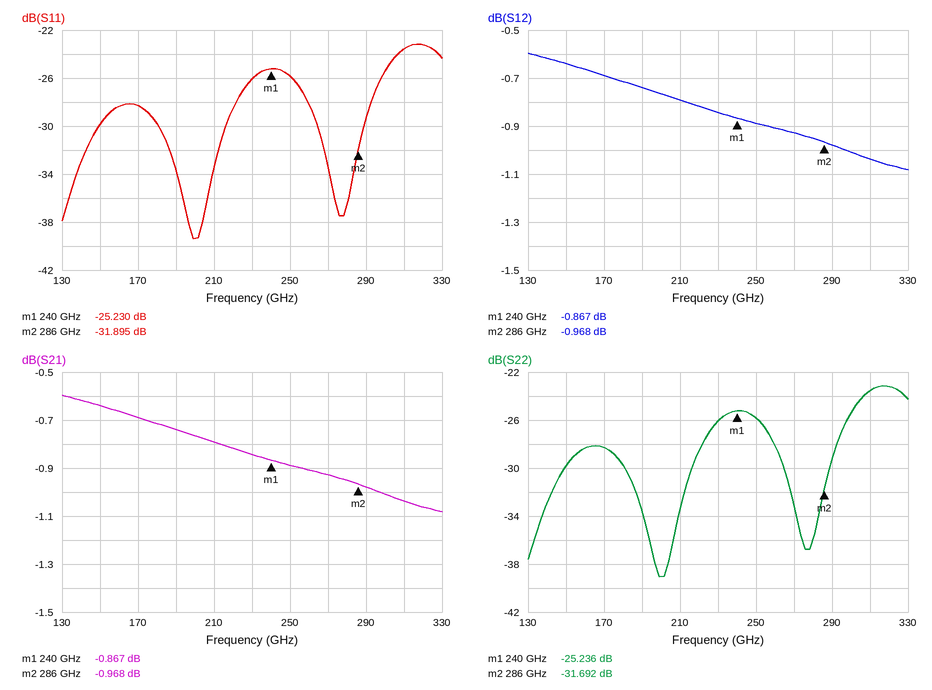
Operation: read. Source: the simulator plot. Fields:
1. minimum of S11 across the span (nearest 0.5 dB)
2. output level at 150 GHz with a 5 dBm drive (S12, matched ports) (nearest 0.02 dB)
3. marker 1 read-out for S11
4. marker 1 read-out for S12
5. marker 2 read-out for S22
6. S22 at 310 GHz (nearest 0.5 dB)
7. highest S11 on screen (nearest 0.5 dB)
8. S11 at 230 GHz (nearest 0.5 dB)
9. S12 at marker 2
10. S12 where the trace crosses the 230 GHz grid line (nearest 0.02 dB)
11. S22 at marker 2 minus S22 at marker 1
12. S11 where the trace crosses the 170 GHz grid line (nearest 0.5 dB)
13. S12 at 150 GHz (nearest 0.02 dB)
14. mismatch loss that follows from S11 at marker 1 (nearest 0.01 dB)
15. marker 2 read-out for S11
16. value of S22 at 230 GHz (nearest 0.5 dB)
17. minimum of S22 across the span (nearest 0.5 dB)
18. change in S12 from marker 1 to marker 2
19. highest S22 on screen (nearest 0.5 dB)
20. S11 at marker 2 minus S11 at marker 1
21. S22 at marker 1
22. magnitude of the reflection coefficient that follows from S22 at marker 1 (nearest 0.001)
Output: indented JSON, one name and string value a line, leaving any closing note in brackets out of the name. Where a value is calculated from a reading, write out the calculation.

{
  "minimum of S11 across the span": "-39.5 dB",
  "output level at 150 GHz with a 5 dBm drive (S12, matched ports)": "5 dBm + (-0.64 dB) = 4.36 dBm",
  "marker 1 read-out for S11": "-25.230 dB",
  "marker 1 read-out for S12": "-0.867 dB",
  "marker 2 read-out for S22": "-31.692 dB",
  "S22 at 310 GHz": "-23.5 dB",
  "highest S11 on screen": "-23.0 dB",
  "S11 at 230 GHz": "-26.0 dB",
  "S12 at marker 2": "-0.968 dB",
  "S12 where the trace crosses the 230 GHz grid line": "-0.84 dB",
  "S22 at marker 2 minus S22 at marker 1": "-31.692 − (-25.236) = -6.456 dB",
  "S11 where the trace crosses the 170 GHz grid line": "-28.5 dB",
  "S12 at 150 GHz": "-0.64 dB",
  "mismatch loss that follows from S11 at marker 1": "−10 log10(1 − 10^(-25.23/10)) ≈ 0.01 dB",
  "marker 2 read-out for S11": "-31.895 dB",
  "value of S22 at 230 GHz": "-26.0 dB",
  "minimum of S22 across the span": "-39.0 dB",
  "change in S12 from marker 1 to marker 2": "-0.968 − (-0.867) = -0.101 dB",
  "highest S22 on screen": "-23.0 dB",
  "S11 at marker 2 minus S11 at marker 1": "-31.895 − (-25.23) = -6.665 dB",
  "S22 at marker 1": "-25.236 dB",
  "magnitude of the reflection coefficient that follows from S22 at marker 1": "10^(-25.236/20) ≈ 0.055"
}
